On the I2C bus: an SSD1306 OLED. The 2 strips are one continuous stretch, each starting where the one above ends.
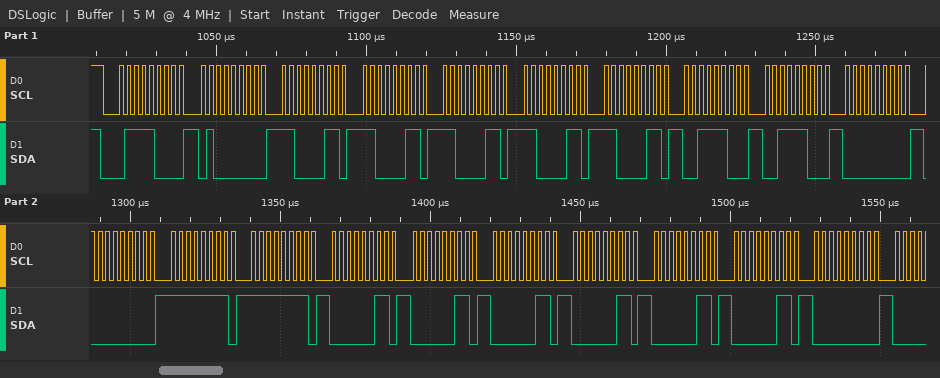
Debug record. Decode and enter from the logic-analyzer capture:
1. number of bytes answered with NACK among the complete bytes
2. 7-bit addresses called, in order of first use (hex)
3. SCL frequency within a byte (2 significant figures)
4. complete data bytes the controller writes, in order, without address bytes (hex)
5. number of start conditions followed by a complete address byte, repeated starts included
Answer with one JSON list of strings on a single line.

["0", "0x3C", "400 kHz", "40 C3 C3 C3 C3 C3 3C 3C 00 00 FF FF 03 03 03 03 03 03 00", "1"]
